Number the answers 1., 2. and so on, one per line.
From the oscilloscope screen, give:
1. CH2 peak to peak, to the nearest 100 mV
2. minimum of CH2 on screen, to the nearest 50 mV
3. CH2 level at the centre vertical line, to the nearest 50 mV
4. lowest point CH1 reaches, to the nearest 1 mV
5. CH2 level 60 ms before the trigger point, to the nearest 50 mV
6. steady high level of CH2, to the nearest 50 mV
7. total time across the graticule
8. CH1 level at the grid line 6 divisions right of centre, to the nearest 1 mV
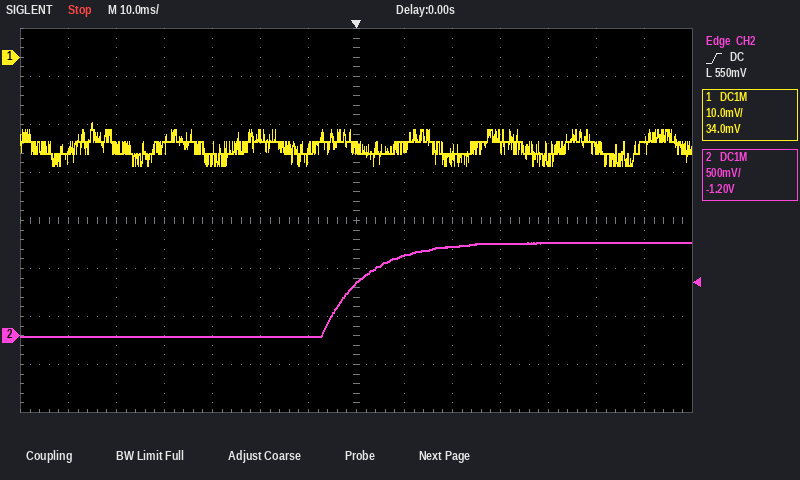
1. 1.00 V
2. 0 mV
3. 550 mV
4. -23 mV
5. 0 mV
6. 950 mV
7. 140 ms
8. -17 mV
